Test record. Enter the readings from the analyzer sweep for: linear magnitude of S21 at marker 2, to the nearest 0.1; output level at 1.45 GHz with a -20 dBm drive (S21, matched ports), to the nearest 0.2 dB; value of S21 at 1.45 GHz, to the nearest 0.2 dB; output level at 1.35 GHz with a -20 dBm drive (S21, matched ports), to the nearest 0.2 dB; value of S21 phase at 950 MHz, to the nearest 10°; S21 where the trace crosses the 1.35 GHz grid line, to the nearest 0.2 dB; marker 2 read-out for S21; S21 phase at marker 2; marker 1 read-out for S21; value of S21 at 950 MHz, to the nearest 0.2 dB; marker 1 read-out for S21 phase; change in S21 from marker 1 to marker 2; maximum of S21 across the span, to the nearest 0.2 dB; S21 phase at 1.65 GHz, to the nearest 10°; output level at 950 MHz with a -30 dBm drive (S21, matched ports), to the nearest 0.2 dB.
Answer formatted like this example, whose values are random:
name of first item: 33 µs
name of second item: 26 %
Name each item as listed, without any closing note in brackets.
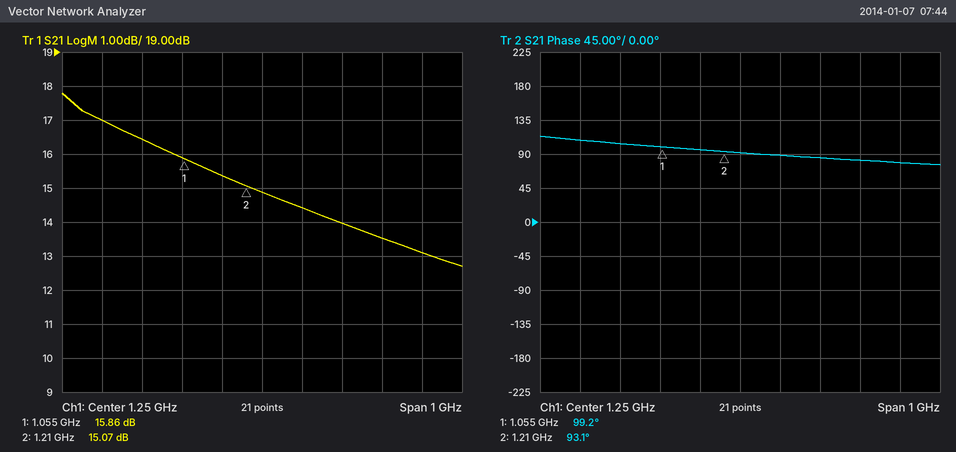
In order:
linear magnitude of S21 at marker 2, to the nearest 0.1: 5.7
output level at 1.45 GHz with a -20 dBm drive (S21, matched ports), to the nearest 0.2 dB: -6.0 dBm
value of S21 at 1.45 GHz, to the nearest 0.2 dB: 14.0 dB
output level at 1.35 GHz with a -20 dBm drive (S21, matched ports), to the nearest 0.2 dB: -5.6 dBm
value of S21 phase at 950 MHz, to the nearest 10°: 100°
S21 where the trace crosses the 1.35 GHz grid line, to the nearest 0.2 dB: 14.4 dB
marker 2 read-out for S21: 15.07 dB
S21 phase at marker 2: 93.1°
marker 1 read-out for S21: 15.86 dB
value of S21 at 950 MHz, to the nearest 0.2 dB: 16.4 dB
marker 1 read-out for S21 phase: 99.2°
change in S21 from marker 1 to marker 2: -0.79 dB
maximum of S21 across the span, to the nearest 0.2 dB: 17.8 dB
S21 phase at 1.65 GHz, to the nearest 10°: 80°
output level at 950 MHz with a -30 dBm drive (S21, matched ports), to the nearest 0.2 dB: -13.6 dBm
